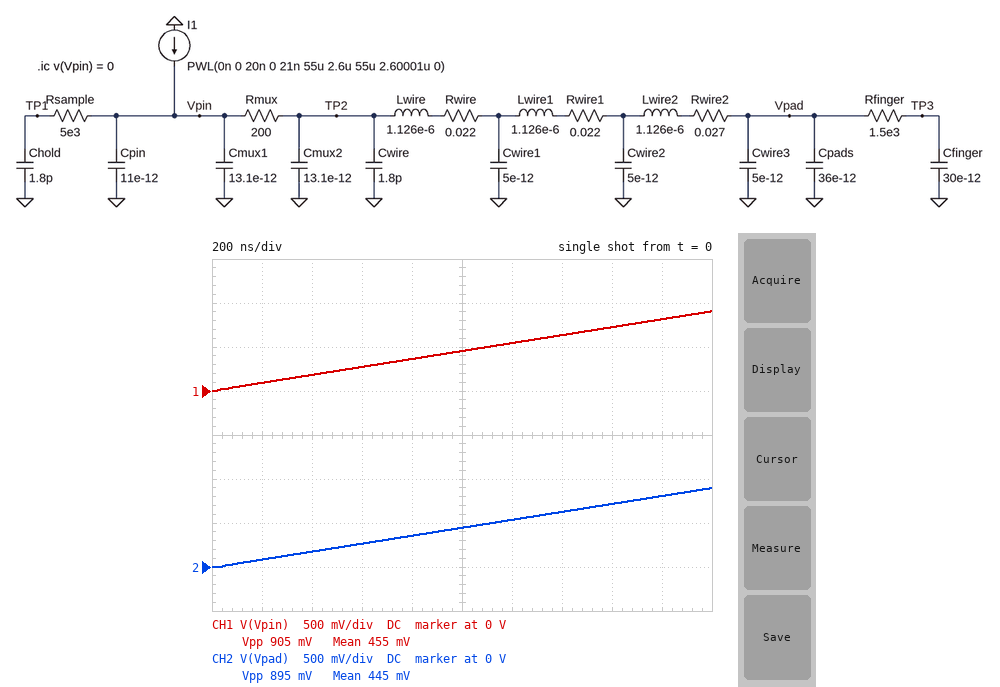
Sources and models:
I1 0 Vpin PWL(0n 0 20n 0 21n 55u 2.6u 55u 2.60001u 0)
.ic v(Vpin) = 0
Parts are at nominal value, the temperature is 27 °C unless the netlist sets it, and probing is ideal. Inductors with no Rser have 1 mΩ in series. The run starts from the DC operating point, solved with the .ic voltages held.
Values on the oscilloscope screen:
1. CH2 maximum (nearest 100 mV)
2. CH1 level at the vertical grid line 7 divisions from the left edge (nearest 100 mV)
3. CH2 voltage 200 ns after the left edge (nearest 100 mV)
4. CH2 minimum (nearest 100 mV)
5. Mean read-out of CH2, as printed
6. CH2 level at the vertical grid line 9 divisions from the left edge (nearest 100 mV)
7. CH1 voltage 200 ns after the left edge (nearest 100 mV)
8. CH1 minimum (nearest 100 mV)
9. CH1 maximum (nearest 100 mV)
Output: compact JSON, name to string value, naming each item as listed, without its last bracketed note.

{"CH2 maximum": "900 mV", "CH1 level at the vertical grid line 7 divisions from the left edge": "600 mV", "CH2 voltage 200 ns after the left edge": "100 mV", "CH2 minimum": "0 V", "Mean read-out of CH2, as printed": "445 mV", "CH2 level at the vertical grid line 9 divisions from the left edge": "800 mV", "CH1 voltage 200 ns after the left edge": "100 mV", "CH1 minimum": "0 V", "CH1 maximum": "900 mV"}
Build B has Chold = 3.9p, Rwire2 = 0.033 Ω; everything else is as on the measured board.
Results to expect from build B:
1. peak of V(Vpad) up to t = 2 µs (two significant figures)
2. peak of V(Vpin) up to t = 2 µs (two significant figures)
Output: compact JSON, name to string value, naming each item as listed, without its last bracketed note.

{"peak of V(Vpad) up to t = 2 µs": "880 mV", "peak of V(Vpin) up to t = 2 µs": "890 mV"}
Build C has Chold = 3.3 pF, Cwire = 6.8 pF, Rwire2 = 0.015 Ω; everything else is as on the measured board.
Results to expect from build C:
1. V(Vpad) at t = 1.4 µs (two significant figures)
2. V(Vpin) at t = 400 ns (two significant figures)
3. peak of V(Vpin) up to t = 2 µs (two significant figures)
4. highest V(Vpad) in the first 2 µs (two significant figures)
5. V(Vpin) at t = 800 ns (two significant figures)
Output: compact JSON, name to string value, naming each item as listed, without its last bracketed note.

{"V(Vpad) at t = 1.4 µs": "590 mV", "V(Vpin) at t = 400 ns": "170 mV", "peak of V(Vpin) up to t = 2 µs": "860 mV", "highest V(Vpad) in the first 2 µs": "850 mV", "V(Vpin) at t = 800 ns": "350 mV"}
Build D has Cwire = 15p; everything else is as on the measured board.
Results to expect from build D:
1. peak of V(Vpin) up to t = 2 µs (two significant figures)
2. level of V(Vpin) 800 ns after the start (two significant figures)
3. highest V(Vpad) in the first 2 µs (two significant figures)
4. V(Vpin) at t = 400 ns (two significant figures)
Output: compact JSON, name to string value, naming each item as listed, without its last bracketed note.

{"peak of V(Vpin) up to t = 2 µs": "820 mV", "level of V(Vpin) 800 ns after the start": "330 mV", "highest V(Vpad) in the first 2 µs": "810 mV", "V(Vpin) at t = 400 ns": "170 mV"}
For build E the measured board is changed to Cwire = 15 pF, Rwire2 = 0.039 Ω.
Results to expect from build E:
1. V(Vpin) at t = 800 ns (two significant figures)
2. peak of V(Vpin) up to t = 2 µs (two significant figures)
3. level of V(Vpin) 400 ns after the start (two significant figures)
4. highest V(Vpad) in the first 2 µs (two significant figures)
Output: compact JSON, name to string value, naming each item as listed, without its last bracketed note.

{"V(Vpin) at t = 800 ns": "330 mV", "peak of V(Vpin) up to t = 2 µs": "820 mV", "level of V(Vpin) 400 ns after the start": "170 mV", "highest V(Vpad) in the first 2 µs": "810 mV"}
